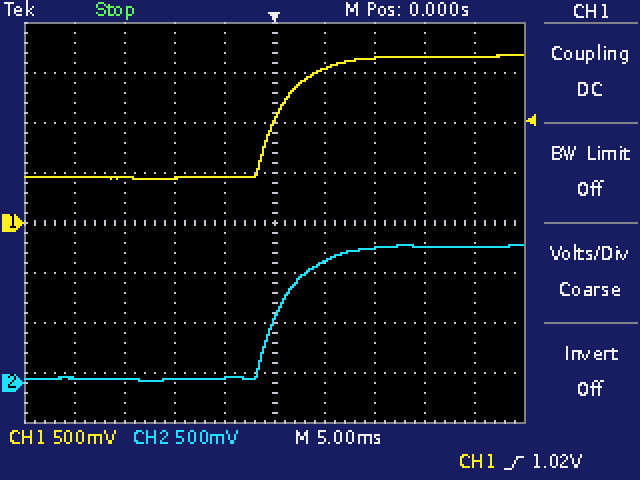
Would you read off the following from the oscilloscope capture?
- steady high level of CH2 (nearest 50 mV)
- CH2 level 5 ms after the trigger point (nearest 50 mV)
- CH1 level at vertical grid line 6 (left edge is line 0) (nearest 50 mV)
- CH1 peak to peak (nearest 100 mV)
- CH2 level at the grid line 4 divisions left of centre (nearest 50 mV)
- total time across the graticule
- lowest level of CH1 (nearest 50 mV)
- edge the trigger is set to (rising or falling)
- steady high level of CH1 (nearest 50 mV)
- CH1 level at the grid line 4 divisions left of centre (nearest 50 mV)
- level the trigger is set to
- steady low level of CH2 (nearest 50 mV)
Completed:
1.35 V
1.20 V
1.55 V
1.20 V
50 mV
50 ms
450 mV
rising
1.65 V
450 mV
1.02 V
50 mV
